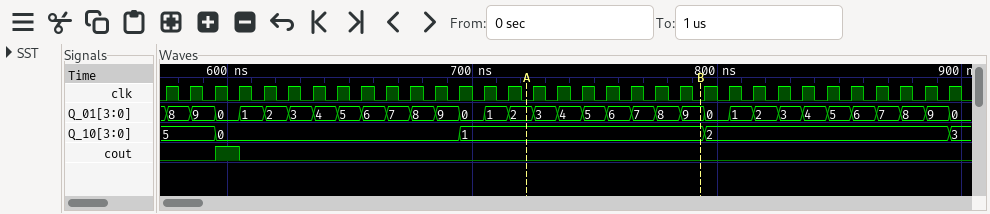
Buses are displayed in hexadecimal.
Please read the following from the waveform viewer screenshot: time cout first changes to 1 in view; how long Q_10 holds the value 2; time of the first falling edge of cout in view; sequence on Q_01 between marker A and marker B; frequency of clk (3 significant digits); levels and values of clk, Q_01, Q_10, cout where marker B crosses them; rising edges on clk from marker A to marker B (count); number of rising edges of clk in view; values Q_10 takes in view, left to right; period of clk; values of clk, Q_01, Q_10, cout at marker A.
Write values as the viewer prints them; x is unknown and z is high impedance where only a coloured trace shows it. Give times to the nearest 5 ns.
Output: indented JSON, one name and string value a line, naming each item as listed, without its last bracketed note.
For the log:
{
  "time cout first changes to 1 in view": "595 ns",
  "how long Q_10 holds the value 2": "100 ns",
  "time of the first falling edge of cout in view": "605 ns",
  "sequence on Q_01 between marker A and marker B": "2, 3, 4, 5, 6, 7, 8, 9",
  "frequency of clk": "100 MHz",
  "levels and values of clk, Q_01, Q_10, cout where marker B crosses them": "clk=0, Q_01=9, Q_10=1, cout=0",
  "rising edges on clk from marker A to marker B": "7",
  "number of rising edges of clk in view": "33",
  "values Q_10 takes in view, left to right": "5, 0, 1, 2, 3",
  "period of clk": "10 ns",
  "values of clk, Q_01, Q_10, cout at marker A": "clk=0, Q_01=2, Q_10=1, cout=0"
}
